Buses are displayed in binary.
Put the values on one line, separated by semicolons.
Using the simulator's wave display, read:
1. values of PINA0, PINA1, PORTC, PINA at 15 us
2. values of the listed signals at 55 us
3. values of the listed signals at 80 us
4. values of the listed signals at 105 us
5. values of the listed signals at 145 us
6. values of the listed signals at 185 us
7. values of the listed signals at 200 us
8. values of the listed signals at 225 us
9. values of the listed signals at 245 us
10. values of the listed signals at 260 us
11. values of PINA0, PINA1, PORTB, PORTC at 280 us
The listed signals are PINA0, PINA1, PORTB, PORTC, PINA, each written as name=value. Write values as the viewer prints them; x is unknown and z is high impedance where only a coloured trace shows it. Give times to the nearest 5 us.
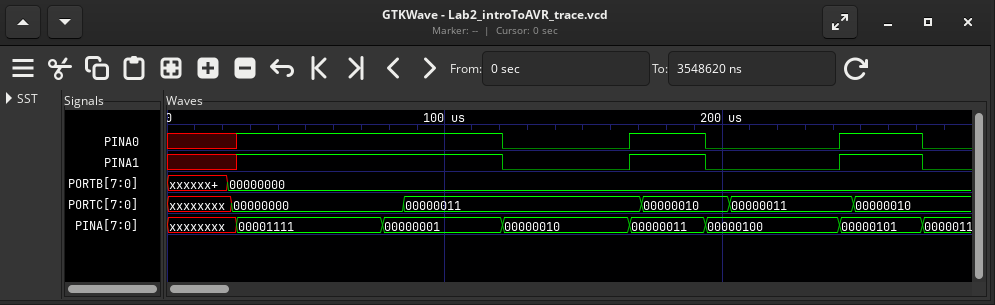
PINA0=x, PINA1=x, PORTC=xxxxxxxx, PINA=xxxxxxxx; PINA0=1, PINA1=1, PORTB=00000000, PORTC=00000000, PINA=00001111; PINA0=1, PINA1=1, PORTB=00000000, PORTC=00000000, PINA=00000001; PINA0=1, PINA1=1, PORTB=00000000, PORTC=00000011, PINA=00000001; PINA0=0, PINA1=0, PORTB=00000000, PORTC=00000011, PINA=00000010; PINA0=1, PINA1=1, PORTB=00000000, PORTC=00000010, PINA=00000011; PINA0=0, PINA1=0, PORTB=00000000, PORTC=00000010, PINA=00000100; PINA0=0, PINA1=0, PORTB=00000000, PORTC=00000011, PINA=00000100; PINA0=1, PINA1=1, PORTB=00000000, PORTC=00000011, PINA=00000101; PINA0=1, PINA1=1, PORTB=00000000, PORTC=00000010, PINA=00000101; PINA0=0, PINA1=0, PORTB=00000000, PORTC=00000010
